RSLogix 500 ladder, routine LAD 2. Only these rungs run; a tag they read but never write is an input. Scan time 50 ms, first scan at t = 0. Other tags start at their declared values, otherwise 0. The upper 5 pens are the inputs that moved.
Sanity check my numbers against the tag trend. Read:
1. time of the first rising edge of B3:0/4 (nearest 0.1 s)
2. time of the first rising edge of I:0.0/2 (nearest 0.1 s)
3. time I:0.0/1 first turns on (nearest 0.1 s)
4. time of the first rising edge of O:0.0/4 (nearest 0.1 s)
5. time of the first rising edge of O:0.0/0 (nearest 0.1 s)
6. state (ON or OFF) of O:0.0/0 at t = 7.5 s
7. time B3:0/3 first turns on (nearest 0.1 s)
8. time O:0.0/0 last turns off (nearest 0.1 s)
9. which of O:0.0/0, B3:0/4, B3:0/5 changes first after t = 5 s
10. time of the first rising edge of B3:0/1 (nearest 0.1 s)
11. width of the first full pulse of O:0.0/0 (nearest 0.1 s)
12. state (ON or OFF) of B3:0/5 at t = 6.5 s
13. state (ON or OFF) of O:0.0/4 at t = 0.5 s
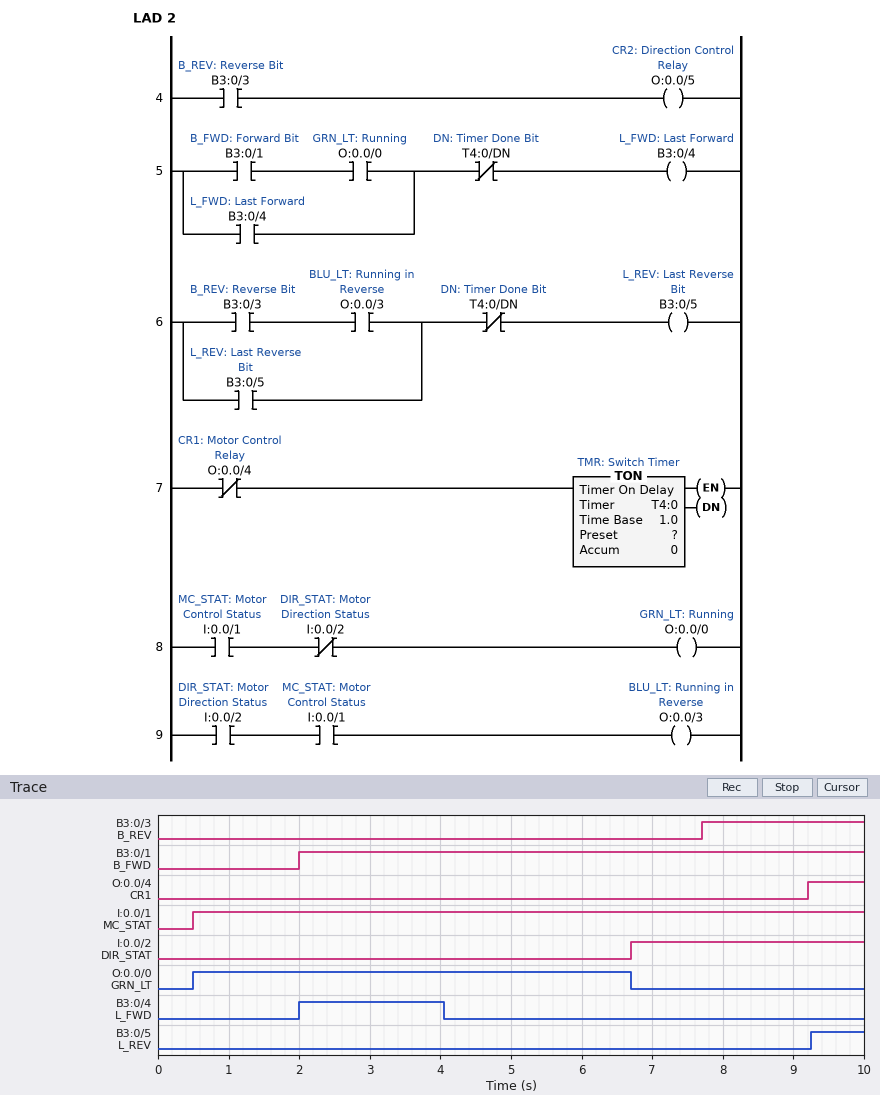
2.0 s
6.7 s
0.5 s
9.2 s
0.5 s
OFF
7.7 s
6.7 s
O:0.0/0
2.0 s
6.2 s
OFF
OFF
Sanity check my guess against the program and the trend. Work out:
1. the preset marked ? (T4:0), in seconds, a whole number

4 s
